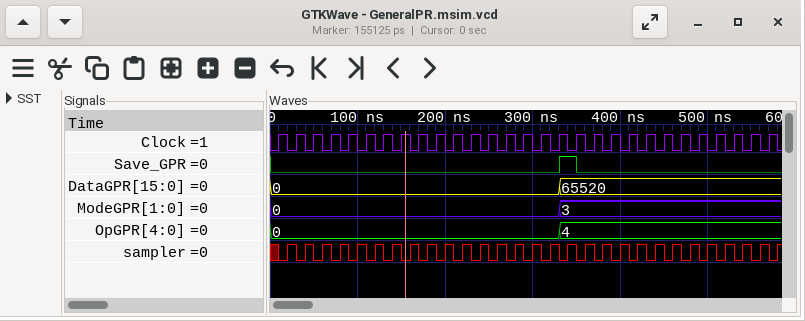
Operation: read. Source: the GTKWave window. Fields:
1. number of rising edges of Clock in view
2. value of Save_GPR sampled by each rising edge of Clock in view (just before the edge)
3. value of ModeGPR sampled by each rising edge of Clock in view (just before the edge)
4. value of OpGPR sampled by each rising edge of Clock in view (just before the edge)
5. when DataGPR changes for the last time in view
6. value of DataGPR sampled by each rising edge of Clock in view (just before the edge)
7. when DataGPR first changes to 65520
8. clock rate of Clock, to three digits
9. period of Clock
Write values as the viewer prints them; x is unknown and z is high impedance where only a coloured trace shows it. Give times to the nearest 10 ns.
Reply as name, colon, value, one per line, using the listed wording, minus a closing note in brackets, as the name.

number of rising edges of Clock in view: 29
value of Save_GPR sampled by each rising edge of Clock in view: 0 0 0 0 0 0 0 0 0 0 0 0 0 0 0 0 0 1 0 0 0 0 0 0 0 0 0 0 0
value of ModeGPR sampled by each rising edge of Clock in view: 0, 0, 0, 0, 0, 0, 0, 0, 0, 0, 0, 0, 0, 0, 0, 0, 0, 3, 3, 3, 3, 3, 3, 3, 3, 3, 3, 3, 3
value of OpGPR sampled by each rising edge of Clock in view: 0, 0, 0, 0, 0, 0, 0, 0, 0, 0, 0, 0, 0, 0, 0, 0, 0, 4, 4, 4, 4, 4, 4, 4, 4, 4, 4, 4, 4
when DataGPR changes for the last time in view: 330 ns
value of DataGPR sampled by each rising edge of Clock in view: 0, 0, 0, 0, 0, 0, 0, 0, 0, 0, 0, 0, 0, 0, 0, 0, 0, 65520, 65520, 65520, 65520, 65520, 65520, 65520, 65520, 65520, 65520, 65520, 65520
when DataGPR first changes to 65520: 330 ns
clock rate of Clock, to three digits: 50.0 MHz
period of Clock: 20 ns
